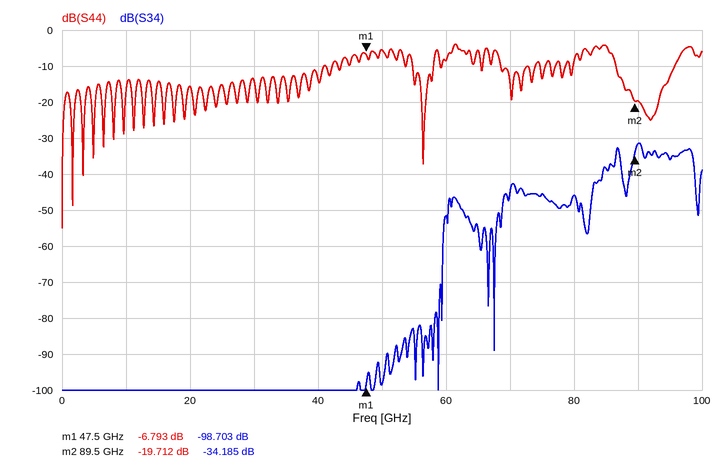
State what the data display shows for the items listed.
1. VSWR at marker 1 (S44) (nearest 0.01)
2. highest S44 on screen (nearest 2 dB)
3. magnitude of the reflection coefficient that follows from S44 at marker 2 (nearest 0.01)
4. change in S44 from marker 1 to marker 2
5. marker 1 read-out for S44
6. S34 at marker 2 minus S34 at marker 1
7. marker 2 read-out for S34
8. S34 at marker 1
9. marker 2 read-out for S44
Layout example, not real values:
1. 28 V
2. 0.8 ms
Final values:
1. 2.69
2. -4 dB
3. 0.10
4. -12.919 dB
5. -6.793 dB
6. 64.518 dB
7. -34.185 dB
8. -98.703 dB
9. -19.712 dB
